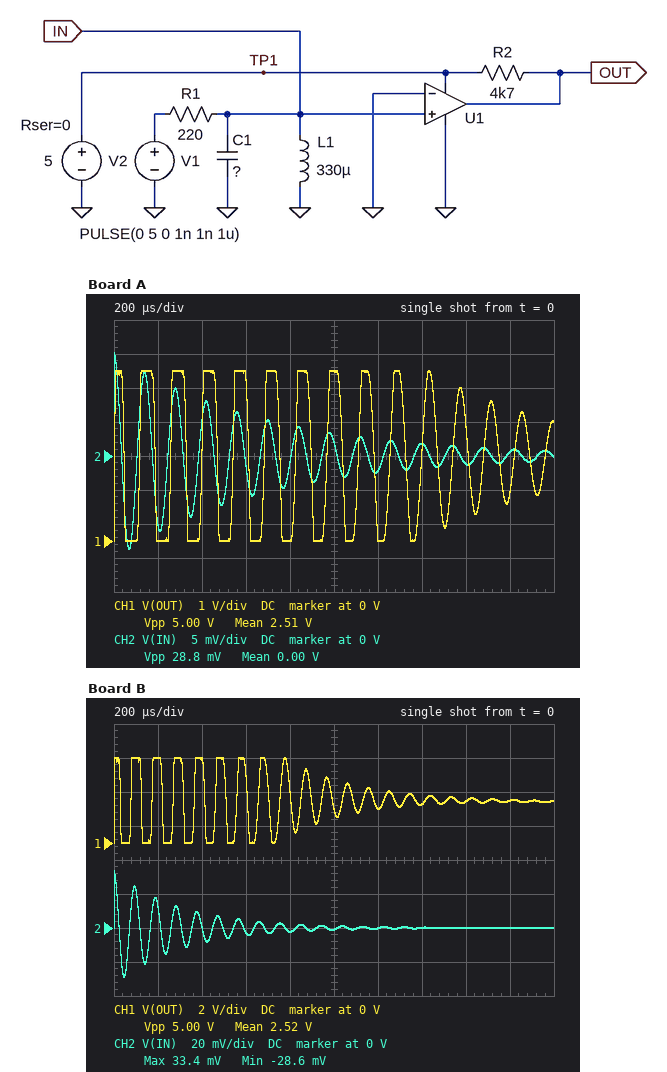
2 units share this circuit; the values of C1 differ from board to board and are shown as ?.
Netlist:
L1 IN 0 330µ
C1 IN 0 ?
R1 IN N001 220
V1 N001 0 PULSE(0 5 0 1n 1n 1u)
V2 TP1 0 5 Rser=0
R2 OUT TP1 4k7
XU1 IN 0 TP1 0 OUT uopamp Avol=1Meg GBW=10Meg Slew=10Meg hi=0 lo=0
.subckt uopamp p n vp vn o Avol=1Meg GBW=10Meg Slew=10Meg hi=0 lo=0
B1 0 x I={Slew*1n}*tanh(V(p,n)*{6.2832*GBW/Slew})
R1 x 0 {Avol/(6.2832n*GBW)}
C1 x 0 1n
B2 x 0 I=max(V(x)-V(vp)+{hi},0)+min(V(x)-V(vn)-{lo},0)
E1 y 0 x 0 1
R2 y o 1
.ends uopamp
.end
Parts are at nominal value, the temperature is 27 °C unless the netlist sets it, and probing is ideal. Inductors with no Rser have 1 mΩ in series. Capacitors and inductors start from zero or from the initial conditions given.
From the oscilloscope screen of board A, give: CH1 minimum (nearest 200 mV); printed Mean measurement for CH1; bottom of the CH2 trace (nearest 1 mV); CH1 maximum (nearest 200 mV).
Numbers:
0 V
2.51 V
-14 mV
5.0 V
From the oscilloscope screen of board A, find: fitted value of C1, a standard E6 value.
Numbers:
1.5 µF
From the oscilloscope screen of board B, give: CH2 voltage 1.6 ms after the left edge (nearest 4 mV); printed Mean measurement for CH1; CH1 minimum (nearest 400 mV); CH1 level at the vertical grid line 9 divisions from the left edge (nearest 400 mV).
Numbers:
0 V
2.52 V
0 V
2.4 V
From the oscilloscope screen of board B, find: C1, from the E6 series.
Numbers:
680 nF
